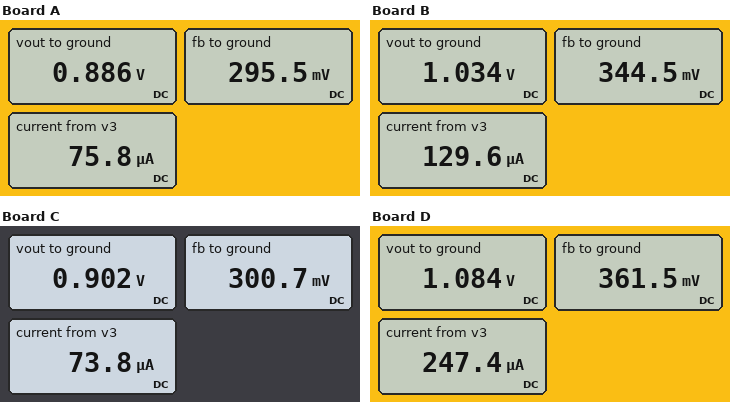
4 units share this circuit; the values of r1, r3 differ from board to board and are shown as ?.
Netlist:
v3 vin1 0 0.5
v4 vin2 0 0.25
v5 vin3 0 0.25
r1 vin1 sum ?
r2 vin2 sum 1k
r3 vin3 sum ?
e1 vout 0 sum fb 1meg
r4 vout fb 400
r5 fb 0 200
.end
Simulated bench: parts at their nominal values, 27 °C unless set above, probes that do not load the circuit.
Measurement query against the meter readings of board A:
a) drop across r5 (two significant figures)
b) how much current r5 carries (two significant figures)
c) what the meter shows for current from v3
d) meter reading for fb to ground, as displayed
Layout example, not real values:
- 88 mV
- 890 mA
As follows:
- 300 mV
- 1.5 mA
- 75.8 µA
- 295.5 mV
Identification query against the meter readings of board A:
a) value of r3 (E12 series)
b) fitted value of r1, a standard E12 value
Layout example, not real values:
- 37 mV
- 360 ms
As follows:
- 1.5 kΩ
- 2.7 kΩ
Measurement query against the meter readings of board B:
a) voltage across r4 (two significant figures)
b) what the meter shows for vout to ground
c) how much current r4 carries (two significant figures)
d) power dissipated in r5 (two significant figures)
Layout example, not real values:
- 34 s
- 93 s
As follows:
- 690 mV
- 1.034 V
- 1.7 mA
- 590 µW
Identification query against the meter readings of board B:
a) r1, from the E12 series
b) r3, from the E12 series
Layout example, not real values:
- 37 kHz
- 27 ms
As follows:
- 1.2 kΩ
- 2.7 kΩ
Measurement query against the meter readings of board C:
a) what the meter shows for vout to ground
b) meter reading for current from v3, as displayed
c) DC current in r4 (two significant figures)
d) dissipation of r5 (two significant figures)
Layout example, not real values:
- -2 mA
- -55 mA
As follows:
- 0.902 V
- 73.8 µA
- 1.5 mA
- 450 µW
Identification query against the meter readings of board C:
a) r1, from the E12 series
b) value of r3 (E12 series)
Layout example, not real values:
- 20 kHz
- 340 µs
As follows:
- 2.7 kΩ
- 2.2 kΩ
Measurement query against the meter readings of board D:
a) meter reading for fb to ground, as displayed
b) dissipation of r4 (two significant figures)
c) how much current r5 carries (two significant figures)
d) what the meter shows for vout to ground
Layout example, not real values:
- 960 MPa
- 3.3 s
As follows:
- 361.5 mV
- 1.3 mW
- 1.8 mA
- 1.084 V
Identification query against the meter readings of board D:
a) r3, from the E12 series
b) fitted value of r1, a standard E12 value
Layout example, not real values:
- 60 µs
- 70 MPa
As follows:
- 820 Ω
- 560 Ω
